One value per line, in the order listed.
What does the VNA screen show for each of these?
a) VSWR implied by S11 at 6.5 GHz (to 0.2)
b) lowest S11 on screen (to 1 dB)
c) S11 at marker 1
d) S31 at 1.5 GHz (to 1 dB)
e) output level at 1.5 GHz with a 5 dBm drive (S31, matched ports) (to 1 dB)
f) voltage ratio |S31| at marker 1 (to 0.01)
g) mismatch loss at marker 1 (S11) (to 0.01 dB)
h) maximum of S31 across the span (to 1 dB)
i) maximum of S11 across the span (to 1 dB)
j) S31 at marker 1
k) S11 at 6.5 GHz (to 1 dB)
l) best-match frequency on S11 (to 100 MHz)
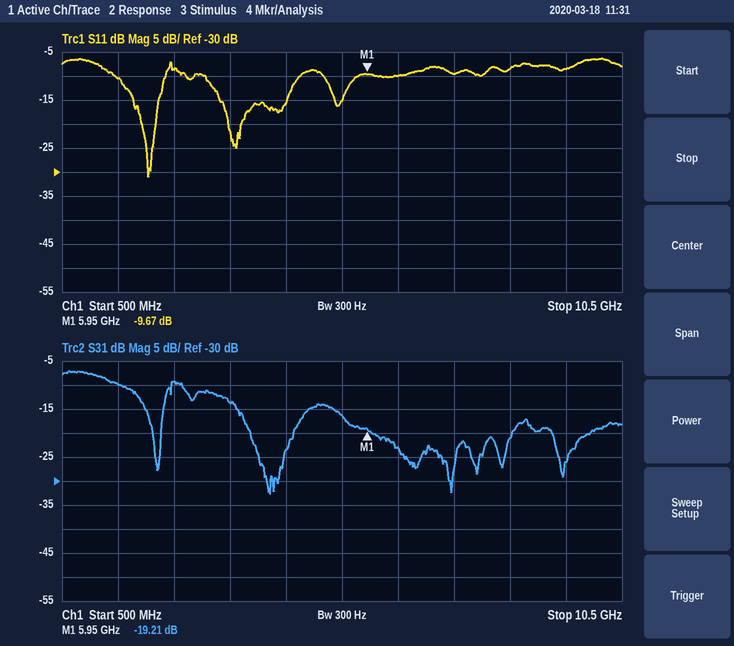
2.0
-31 dB
-9.67 dB
-10 dB
-5 dBm
0.11
0.50 dB
-7 dB
-6 dB
-19.21 dB
-10 dB
2.0 GHz
